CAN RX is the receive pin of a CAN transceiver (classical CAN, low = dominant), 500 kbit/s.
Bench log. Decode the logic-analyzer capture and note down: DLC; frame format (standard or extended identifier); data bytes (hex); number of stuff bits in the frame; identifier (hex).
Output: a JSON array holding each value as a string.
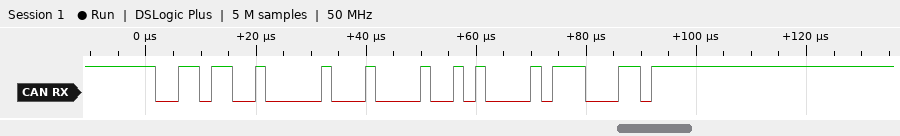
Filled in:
["1", "standard", "09", "1", "0x364"]
